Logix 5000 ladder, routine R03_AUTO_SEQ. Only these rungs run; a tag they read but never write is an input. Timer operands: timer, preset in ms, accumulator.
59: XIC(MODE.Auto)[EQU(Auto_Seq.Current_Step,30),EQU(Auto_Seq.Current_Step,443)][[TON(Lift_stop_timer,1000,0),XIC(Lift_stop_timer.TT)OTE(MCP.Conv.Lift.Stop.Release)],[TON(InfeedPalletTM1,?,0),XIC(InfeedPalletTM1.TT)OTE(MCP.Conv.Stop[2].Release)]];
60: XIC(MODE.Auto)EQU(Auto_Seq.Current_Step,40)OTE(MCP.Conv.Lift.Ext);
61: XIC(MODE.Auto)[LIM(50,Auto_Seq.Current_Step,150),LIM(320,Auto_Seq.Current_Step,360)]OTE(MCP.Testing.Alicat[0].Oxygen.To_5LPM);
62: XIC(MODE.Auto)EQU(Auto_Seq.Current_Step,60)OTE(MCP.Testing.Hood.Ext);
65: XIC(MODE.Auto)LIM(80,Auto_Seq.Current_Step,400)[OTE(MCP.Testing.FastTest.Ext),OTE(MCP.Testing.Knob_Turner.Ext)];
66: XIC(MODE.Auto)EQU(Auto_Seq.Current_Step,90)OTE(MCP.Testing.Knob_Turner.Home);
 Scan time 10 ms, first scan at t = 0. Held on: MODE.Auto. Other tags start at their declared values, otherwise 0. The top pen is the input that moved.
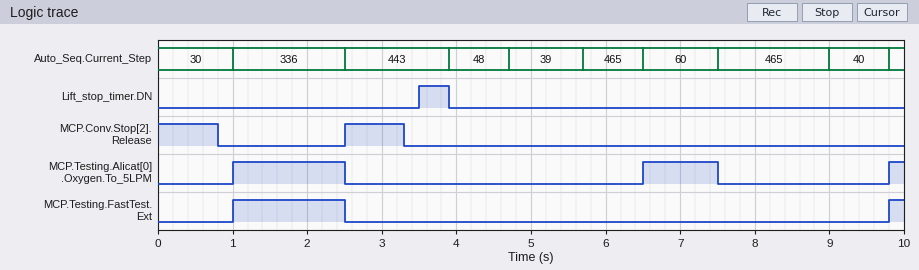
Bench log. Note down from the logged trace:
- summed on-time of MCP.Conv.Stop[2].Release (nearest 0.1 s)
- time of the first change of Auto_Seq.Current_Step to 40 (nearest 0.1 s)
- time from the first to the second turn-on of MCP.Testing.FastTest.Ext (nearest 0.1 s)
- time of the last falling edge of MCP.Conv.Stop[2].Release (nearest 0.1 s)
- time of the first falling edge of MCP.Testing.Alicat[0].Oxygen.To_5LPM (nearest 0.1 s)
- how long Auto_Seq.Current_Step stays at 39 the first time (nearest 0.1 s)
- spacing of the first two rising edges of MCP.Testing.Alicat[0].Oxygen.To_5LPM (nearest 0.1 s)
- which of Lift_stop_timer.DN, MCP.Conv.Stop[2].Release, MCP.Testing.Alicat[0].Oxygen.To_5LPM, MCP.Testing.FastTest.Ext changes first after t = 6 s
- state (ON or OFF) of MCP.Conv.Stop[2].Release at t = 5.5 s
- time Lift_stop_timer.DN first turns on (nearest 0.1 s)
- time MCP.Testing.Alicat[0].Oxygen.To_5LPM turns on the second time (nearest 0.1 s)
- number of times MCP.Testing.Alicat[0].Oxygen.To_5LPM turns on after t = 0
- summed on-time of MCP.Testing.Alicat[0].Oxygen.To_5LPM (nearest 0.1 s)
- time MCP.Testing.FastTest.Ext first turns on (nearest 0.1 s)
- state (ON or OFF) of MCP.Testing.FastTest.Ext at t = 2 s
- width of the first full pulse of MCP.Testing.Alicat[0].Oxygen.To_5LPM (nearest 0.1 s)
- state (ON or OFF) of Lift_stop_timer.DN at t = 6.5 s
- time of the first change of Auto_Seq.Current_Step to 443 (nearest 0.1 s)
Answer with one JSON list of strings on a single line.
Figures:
["1.6 s", "9.0 s", "8.8 s", "3.3 s", "2.5 s", "1.0 s", "5.5 s", "MCP.Testing.Alicat[0].Oxygen.To_5LPM", "OFF", "3.5 s", "6.5 s", "3", "2.7 s", "1.0 s", "ON", "1.5 s", "OFF", "2.5 s"]
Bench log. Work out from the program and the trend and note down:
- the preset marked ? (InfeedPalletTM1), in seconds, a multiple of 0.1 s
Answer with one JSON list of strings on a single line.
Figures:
["0.8 s"]
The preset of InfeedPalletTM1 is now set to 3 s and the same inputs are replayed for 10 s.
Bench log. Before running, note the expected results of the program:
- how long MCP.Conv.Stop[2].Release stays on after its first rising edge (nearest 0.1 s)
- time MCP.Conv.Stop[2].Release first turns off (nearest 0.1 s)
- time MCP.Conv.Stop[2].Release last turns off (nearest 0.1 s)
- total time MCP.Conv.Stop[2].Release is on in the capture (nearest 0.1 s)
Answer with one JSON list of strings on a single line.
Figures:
["1.4 s", "1.0 s", "3.9 s", "2.4 s"]
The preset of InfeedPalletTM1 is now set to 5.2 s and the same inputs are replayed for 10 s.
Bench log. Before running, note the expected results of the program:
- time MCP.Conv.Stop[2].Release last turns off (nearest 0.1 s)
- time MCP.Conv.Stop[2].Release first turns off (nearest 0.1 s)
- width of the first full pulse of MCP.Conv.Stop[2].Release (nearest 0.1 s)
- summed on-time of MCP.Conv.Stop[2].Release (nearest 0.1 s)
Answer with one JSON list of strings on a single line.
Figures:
["3.9 s", "1.0 s", "1.4 s", "2.4 s"]
